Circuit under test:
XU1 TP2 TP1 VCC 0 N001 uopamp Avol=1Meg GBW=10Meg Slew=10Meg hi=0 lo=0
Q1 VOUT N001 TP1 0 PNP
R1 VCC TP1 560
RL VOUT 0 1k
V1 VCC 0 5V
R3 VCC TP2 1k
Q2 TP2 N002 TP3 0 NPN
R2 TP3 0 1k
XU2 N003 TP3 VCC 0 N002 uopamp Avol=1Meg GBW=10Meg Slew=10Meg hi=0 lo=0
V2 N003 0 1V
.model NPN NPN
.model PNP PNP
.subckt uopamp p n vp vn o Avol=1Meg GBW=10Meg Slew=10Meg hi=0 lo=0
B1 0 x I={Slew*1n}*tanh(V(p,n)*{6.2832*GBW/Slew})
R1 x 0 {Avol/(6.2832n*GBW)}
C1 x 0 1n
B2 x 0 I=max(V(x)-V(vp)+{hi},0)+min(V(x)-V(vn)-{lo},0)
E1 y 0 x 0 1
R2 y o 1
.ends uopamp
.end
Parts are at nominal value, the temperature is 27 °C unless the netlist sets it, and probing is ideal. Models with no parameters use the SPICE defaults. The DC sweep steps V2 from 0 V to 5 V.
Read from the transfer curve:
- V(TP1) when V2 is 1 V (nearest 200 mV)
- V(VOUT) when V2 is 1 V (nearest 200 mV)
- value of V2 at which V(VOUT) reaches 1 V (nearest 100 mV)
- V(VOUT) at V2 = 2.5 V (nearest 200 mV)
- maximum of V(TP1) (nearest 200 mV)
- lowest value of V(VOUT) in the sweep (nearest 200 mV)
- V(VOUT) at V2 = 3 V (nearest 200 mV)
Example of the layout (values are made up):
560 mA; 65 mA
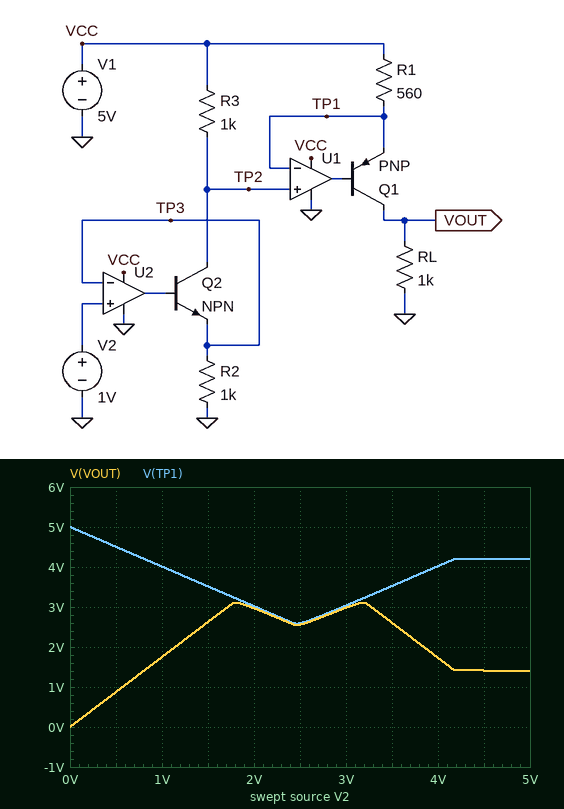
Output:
4.0 V; 1.8 V; 600 mV; 2.6 V; 5.0 V; 0 V; 3.0 V
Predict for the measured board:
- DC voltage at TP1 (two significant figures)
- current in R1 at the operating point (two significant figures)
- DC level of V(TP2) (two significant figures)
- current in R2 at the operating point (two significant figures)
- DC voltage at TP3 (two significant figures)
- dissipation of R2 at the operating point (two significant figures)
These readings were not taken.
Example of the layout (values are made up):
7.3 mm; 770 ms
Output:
4.0 V; 1.8 mA; 4.0 V; 1.0 mA; 1.0 V; 1.0 mW
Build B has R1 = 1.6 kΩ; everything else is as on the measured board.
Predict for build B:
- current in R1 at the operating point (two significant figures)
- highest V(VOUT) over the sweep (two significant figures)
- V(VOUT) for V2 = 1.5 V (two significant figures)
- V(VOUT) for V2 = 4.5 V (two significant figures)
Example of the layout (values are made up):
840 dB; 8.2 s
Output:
620 µA; 1.5 V; 920 mV; 490 mV
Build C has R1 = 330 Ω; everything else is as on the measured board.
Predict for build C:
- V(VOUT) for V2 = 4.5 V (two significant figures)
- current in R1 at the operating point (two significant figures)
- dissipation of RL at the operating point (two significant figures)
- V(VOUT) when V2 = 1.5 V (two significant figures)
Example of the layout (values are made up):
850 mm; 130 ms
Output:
2.4 V; 3.0 mA; 8.8 mW; 3.5 V
